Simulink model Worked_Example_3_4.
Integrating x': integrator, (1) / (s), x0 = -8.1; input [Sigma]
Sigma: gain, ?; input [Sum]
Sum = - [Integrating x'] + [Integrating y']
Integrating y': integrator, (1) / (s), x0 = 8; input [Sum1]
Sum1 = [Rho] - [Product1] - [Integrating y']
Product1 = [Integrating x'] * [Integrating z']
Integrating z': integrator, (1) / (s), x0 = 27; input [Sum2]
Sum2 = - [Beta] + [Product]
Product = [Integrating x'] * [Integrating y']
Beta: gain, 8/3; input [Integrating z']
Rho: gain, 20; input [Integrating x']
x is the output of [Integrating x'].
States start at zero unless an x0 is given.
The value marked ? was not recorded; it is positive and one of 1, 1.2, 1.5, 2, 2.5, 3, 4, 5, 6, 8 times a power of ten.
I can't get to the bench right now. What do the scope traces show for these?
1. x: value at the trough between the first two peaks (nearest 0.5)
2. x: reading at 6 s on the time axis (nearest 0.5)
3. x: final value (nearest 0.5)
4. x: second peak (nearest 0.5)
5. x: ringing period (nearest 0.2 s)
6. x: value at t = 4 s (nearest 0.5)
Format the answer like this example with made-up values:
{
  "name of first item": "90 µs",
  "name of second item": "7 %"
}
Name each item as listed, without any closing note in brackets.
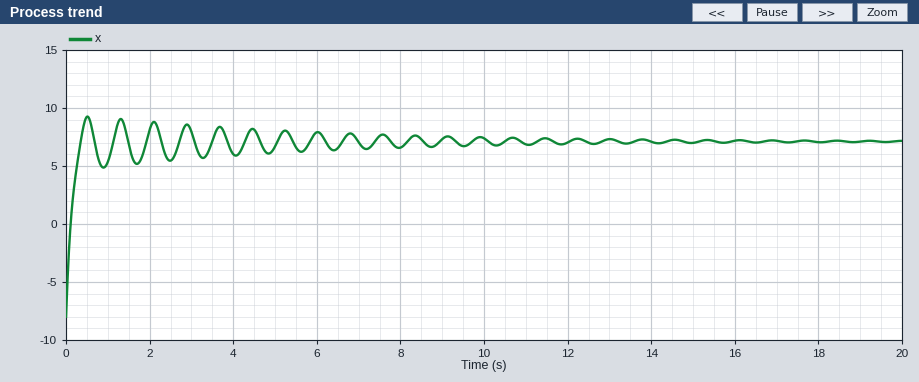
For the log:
{
  "x: value at the trough between the first two peaks": "5.0",
  "x: reading at 6 s on the time axis": "8.0",
  "x: final value": "7.0",
  "x: second peak": "9.0",
  "x: ringing period": "0.8 s",
  "x: value at t = 4 s": "6.0"
}
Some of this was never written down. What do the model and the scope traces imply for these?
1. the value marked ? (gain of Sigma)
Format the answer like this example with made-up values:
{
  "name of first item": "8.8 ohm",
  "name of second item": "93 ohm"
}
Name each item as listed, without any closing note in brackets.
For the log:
{
  "the value marked ?": "6"
}
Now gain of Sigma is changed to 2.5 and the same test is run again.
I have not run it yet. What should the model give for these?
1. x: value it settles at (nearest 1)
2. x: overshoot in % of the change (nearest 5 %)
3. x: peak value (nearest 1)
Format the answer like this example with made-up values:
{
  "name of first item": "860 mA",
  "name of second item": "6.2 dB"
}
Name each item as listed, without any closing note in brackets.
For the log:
{
  "x: value it settles at": "7",
  "x: overshoot in % of the change": "20 %",
  "x: peak value": "10"
}
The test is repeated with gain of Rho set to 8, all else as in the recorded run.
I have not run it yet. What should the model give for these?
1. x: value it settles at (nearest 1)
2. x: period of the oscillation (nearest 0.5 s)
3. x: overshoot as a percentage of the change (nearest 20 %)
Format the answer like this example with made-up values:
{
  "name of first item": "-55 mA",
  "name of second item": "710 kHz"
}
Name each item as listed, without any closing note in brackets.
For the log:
{
  "x: value it settles at": "-4",
  "x: period of the oscillation": "3.0 s",
  "x: overshoot as a percentage of the change": "260 %"
}
